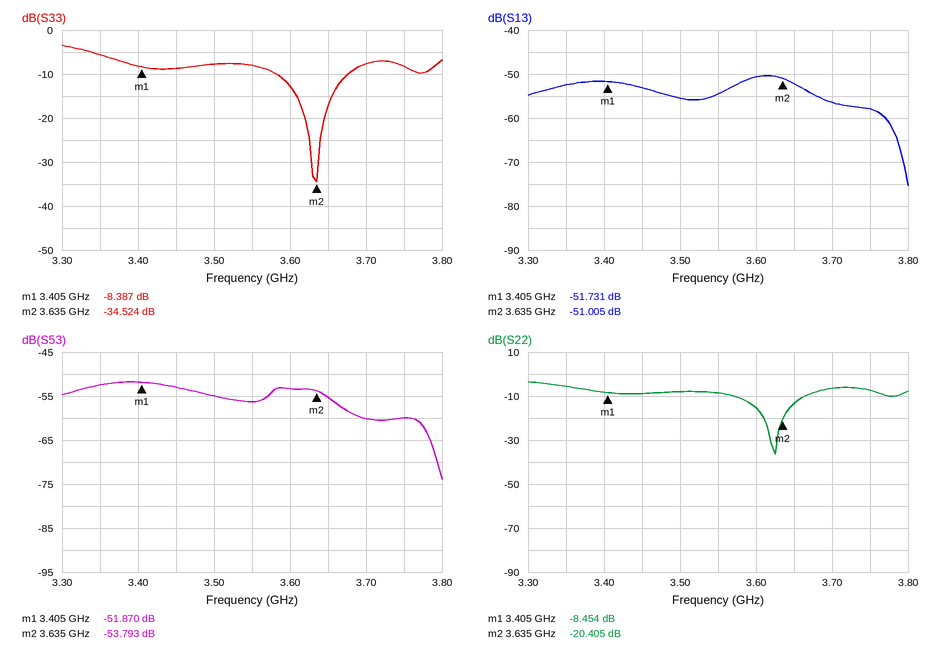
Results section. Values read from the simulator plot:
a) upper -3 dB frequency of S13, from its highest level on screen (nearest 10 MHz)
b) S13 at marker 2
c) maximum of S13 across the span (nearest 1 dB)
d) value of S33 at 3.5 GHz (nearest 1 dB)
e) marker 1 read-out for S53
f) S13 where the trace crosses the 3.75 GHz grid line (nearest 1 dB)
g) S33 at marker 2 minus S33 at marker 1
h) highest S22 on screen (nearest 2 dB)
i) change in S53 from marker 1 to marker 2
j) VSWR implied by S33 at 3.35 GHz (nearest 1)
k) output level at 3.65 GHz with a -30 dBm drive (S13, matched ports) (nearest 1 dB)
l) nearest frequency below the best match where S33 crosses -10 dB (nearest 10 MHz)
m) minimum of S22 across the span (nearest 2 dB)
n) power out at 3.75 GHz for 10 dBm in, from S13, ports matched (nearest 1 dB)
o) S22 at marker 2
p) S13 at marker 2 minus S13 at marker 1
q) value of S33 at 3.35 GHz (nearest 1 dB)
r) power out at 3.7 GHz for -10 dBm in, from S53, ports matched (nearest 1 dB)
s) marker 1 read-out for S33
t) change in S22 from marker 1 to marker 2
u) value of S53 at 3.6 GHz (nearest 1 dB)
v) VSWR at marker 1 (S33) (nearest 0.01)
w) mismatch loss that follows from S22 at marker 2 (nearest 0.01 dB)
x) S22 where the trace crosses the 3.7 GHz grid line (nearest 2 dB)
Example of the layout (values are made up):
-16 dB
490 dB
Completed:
3.66 GHz
-51.005 dB
-50 dB
-8 dB
-51.870 dB
-58 dB
-26.137 dB
-4 dB
-1.923 dB
3
-82 dBm
3.58 GHz
-36 dB
-48 dBm
-20.405 dB
0.726 dB
-6 dB
-70 dBm
-8.387 dB
-11.951 dB
-53 dB
2.23
0.04 dB
-6 dB
